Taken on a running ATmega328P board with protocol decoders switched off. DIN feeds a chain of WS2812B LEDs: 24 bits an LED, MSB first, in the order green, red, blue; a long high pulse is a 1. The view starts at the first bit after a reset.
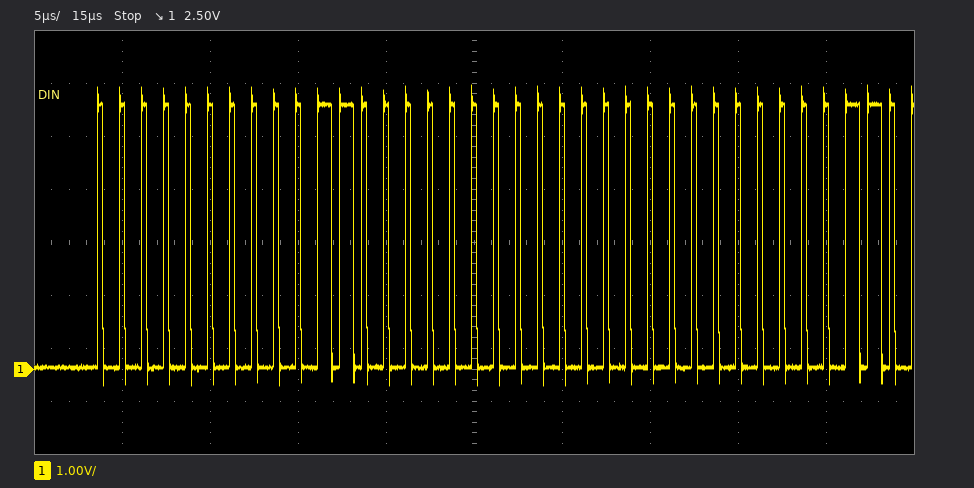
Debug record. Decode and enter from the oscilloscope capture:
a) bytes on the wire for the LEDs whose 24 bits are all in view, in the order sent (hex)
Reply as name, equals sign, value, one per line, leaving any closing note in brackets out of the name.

bytes on the wire for the LEDs whose 24 bits are all in view, in the order sent = 00 30 00
